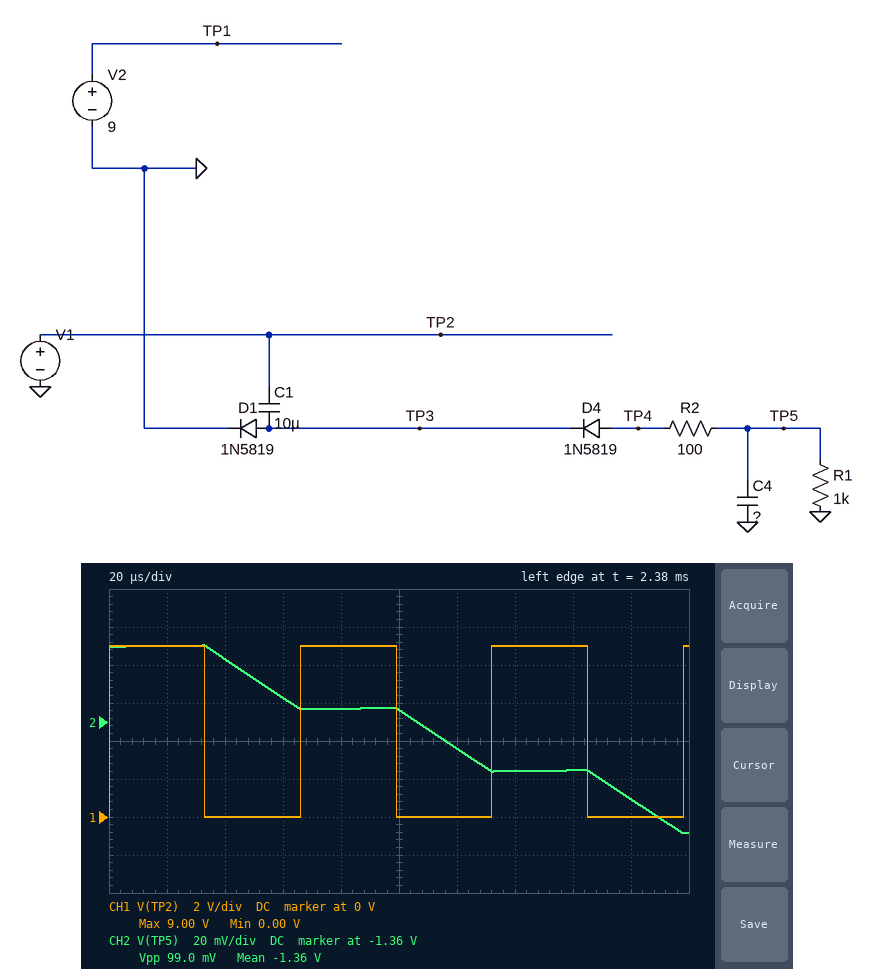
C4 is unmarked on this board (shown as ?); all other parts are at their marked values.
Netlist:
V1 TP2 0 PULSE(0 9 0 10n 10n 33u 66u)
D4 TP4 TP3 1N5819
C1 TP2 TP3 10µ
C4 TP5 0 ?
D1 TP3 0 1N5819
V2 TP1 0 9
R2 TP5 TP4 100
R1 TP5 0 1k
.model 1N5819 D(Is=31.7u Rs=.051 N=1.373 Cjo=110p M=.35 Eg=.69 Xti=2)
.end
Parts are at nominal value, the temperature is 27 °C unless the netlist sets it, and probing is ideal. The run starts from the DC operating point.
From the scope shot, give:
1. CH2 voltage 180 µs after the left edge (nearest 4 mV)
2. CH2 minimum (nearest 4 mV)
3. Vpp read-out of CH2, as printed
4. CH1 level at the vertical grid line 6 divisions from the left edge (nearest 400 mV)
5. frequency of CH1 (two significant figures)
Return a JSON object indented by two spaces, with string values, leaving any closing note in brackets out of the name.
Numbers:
{
  "CH2 voltage 180 µs after the left edge": "-1.400 V",
  "CH2 minimum": "-1.420 V",
  "Vpp read-out of CH2, as printed": "99.0 mV",
  "CH1 level at the vertical grid line 6 divisions from the left edge": "0 V",
  "frequency of CH1": "15 kHz"
}
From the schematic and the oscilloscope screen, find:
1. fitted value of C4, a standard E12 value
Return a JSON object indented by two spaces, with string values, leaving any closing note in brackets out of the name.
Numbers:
{
  "fitted value of C4, a standard E12 value": "68 µF"
}
